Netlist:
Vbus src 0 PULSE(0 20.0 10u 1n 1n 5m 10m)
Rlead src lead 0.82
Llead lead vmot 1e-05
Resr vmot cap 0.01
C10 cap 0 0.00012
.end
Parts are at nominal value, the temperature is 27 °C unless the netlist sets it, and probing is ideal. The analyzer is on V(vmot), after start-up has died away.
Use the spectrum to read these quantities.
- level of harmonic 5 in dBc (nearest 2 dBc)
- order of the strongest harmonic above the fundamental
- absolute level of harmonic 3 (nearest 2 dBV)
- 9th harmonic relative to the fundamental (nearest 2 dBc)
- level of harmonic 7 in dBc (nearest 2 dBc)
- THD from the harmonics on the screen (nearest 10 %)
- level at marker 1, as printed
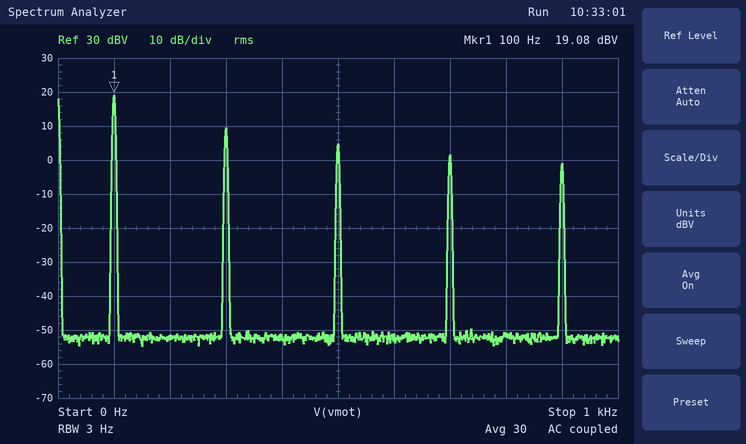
-14 dBc
3
10 dBV
-20 dBc
-18 dBc
40 %
19.08 dBV
